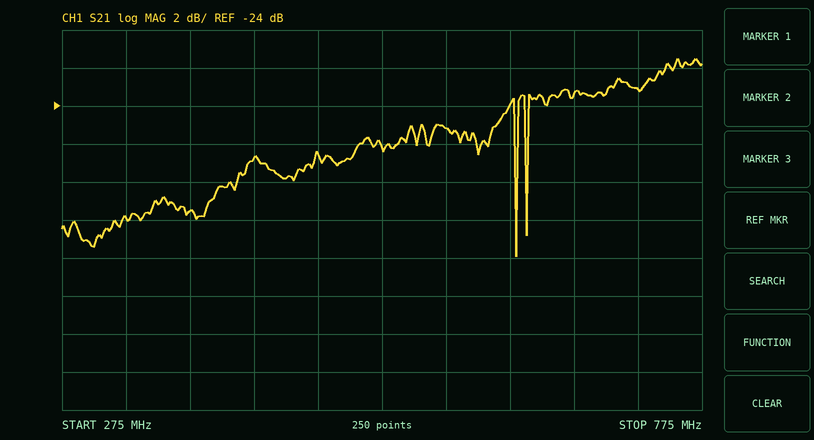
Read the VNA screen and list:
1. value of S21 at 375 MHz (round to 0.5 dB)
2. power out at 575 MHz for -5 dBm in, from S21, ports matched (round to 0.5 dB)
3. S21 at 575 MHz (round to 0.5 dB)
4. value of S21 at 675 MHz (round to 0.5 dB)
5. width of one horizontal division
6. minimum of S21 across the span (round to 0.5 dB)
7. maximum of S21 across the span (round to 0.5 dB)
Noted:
-29.5 dB
-30.0 dBm
-25.0 dB
-23.5 dB
50 MHz
-32.0 dB
-21.5 dB
